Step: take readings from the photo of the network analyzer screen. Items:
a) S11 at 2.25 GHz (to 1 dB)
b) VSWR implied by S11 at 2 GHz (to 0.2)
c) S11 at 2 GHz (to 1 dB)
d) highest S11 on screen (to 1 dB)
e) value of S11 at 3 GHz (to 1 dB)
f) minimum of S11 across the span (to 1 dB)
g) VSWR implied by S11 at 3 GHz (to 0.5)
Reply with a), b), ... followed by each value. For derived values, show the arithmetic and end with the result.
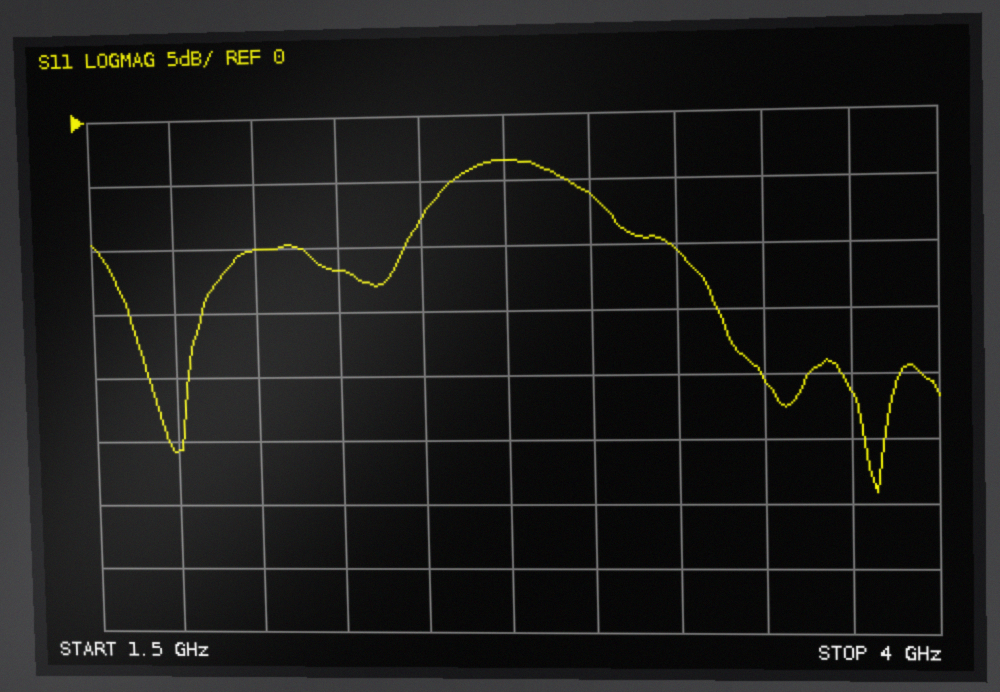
a) -12 dB
b) |Γ| = 10^(-10/20) = 0.3162; VSWR = (1 + 0.3162)/(1 − 0.3162) ≈ 1.92, so 2.0 to the nearest 0.2
c) -10 dB
d) -3 dB
e) -6 dB
f) -29 dB
g) |Γ| = 10^(-6/20) = 0.5012; VSWR = (1 + 0.5012)/(1 − 0.5012) ≈ 3.0
